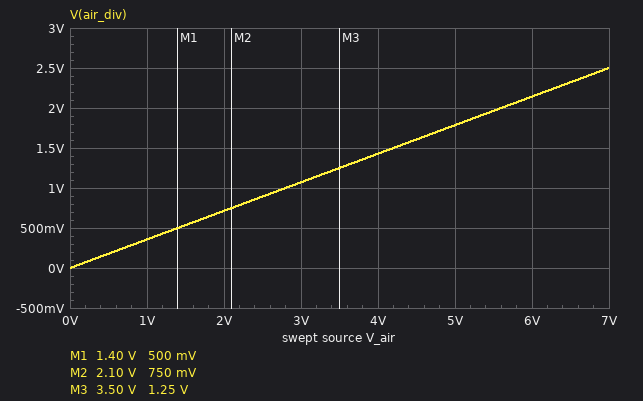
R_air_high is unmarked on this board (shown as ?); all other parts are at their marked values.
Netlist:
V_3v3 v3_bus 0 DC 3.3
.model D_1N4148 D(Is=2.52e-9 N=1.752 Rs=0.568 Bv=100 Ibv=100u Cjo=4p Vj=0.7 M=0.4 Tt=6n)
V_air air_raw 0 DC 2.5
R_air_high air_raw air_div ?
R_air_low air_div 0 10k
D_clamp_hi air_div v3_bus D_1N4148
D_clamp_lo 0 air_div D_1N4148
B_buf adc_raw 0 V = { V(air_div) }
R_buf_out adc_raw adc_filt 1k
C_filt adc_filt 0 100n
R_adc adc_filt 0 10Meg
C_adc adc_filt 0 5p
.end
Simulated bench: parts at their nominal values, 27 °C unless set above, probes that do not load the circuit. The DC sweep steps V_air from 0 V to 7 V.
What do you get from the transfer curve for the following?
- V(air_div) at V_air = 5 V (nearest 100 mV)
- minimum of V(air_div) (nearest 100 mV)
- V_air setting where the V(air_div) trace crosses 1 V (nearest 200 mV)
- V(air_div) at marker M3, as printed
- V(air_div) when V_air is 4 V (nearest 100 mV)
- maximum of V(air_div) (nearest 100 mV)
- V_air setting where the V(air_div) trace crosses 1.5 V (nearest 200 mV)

1.8 V
0 V
2.8 V
1.25 V
1.4 V
2.5 V
4.2 V
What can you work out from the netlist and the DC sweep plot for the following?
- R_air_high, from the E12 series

18 kΩ
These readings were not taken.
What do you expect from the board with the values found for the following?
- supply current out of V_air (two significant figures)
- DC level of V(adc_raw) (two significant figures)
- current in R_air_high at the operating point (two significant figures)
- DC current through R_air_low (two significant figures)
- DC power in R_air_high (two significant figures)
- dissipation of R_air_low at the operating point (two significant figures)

89 µA
890 mV
89 µA
89 µA
140 µW
80 µW
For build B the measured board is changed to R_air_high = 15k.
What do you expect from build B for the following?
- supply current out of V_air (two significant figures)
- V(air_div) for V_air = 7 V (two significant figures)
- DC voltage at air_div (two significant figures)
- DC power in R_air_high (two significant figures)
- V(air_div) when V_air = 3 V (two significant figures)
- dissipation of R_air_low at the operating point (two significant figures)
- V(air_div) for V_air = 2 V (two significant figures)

100 µA
2.8 V
1.0 V
150 µW
1.2 V
100 µW
800 mV
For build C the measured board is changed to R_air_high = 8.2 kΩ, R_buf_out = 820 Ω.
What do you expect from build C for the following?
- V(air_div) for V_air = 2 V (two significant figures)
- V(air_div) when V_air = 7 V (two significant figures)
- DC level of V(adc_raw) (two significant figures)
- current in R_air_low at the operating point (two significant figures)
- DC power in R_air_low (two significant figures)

1.1 V
3.7 V
1.4 V
140 µA
190 µW
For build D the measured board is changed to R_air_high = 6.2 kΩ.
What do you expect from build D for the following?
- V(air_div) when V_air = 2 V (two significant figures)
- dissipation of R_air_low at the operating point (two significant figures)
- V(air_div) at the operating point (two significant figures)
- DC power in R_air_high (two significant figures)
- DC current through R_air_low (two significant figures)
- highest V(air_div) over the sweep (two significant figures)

1.2 V
240 µW
1.5 V
150 µW
150 µA
3.8 V
